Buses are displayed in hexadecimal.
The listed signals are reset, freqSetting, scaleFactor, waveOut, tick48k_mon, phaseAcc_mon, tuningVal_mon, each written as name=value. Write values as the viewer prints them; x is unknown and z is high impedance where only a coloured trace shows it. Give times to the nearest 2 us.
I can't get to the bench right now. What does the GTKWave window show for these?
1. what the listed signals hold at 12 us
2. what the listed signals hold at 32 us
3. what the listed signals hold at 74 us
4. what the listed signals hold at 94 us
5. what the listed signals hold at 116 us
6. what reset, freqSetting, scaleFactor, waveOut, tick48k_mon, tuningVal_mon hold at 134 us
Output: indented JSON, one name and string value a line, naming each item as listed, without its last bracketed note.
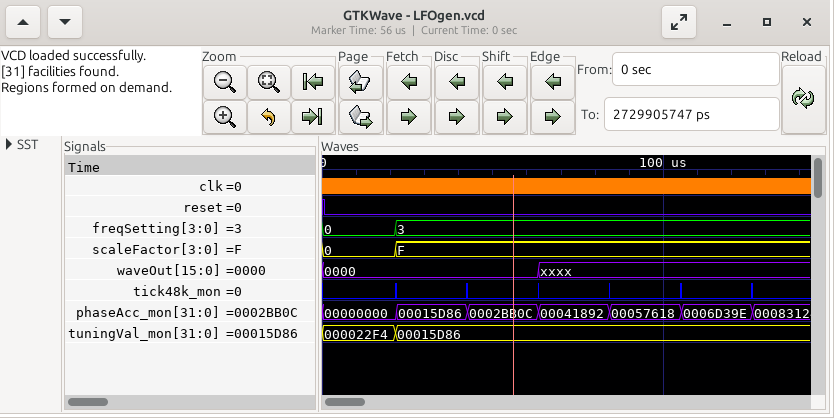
{
  "what the listed signals hold at 12 us": "reset=0, freqSetting=0, scaleFactor=0, waveOut=0000, tick48k_mon=0, phaseAcc_mon=00000000, tuningVal_mon=000022F4",
  "what the listed signals hold at 32 us": "reset=0, freqSetting=3, scaleFactor=F, waveOut=0000, tick48k_mon=0, phaseAcc_mon=00015D86, tuningVal_mon=00015D86",
  "what the listed signals hold at 74 us": "reset=0, freqSetting=3, scaleFactor=F, waveOut=xxxx, tick48k_mon=0, phaseAcc_mon=00041892, tuningVal_mon=00015D86",
  "what the listed signals hold at 94 us": "reset=0, freqSetting=3, scaleFactor=F, waveOut=xxxx, tick48k_mon=0, phaseAcc_mon=00057618, tuningVal_mon=00015D86",
  "what the listed signals hold at 116 us": "reset=0, freqSetting=3, scaleFactor=F, waveOut=xxxx, tick48k_mon=0, phaseAcc_mon=0006D39E, tuningVal_mon=00015D86",
  "what reset, freqSetting, scaleFactor, waveOut, tick48k_mon, tuningVal_mon hold at 134 us": "reset=0, freqSetting=3, scaleFactor=F, waveOut=xxxx, tick48k_mon=0, tuningVal_mon=00015D86"
}
